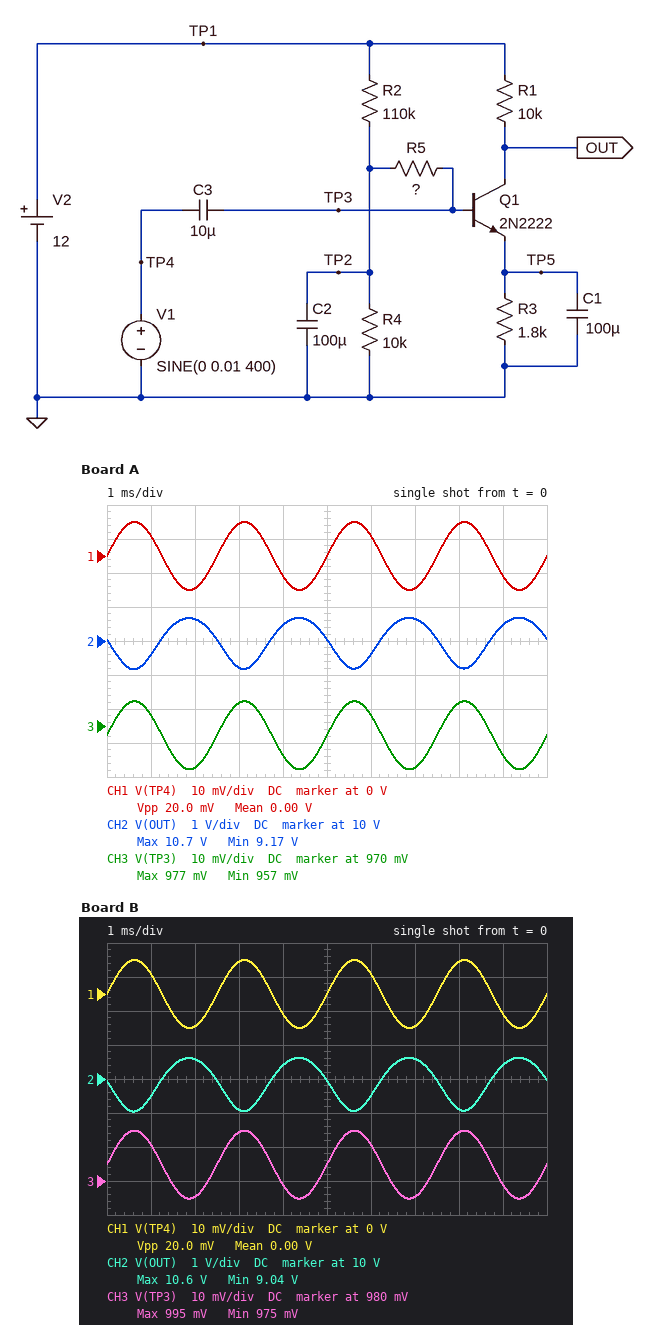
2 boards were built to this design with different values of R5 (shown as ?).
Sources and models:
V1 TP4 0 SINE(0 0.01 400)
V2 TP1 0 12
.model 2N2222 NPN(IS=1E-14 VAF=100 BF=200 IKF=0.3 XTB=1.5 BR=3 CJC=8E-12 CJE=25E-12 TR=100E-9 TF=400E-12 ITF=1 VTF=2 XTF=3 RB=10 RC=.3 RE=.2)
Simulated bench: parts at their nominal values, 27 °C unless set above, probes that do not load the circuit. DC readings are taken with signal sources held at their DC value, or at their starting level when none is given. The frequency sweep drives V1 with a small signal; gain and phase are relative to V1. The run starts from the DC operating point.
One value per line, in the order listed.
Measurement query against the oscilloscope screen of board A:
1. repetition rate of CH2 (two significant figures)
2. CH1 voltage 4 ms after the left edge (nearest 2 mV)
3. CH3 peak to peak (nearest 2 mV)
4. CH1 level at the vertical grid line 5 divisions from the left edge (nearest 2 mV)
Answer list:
400 Hz
-6 mV
20 mV
0 V
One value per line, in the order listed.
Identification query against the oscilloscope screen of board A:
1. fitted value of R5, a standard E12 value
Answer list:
27 kΩ
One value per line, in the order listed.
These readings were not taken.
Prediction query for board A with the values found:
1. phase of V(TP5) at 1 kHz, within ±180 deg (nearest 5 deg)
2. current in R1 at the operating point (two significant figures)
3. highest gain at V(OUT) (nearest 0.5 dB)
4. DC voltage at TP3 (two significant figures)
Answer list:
-90 deg
200 µA
37.5 dB
970 mV
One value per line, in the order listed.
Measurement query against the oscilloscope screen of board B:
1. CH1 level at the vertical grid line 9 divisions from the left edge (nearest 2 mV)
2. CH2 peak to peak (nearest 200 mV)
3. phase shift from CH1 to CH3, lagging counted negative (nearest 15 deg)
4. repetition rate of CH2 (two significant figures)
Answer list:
-6 mV
1.6 V
0 deg
400 Hz
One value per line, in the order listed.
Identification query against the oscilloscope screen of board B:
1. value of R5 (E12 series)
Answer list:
6.8 kΩ
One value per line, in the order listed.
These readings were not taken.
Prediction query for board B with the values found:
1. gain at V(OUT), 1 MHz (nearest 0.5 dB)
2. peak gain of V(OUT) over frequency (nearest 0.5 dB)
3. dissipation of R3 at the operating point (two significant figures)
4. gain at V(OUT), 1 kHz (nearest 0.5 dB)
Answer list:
37.5 dB
38.0 dB
77 µW
38.0 dB
